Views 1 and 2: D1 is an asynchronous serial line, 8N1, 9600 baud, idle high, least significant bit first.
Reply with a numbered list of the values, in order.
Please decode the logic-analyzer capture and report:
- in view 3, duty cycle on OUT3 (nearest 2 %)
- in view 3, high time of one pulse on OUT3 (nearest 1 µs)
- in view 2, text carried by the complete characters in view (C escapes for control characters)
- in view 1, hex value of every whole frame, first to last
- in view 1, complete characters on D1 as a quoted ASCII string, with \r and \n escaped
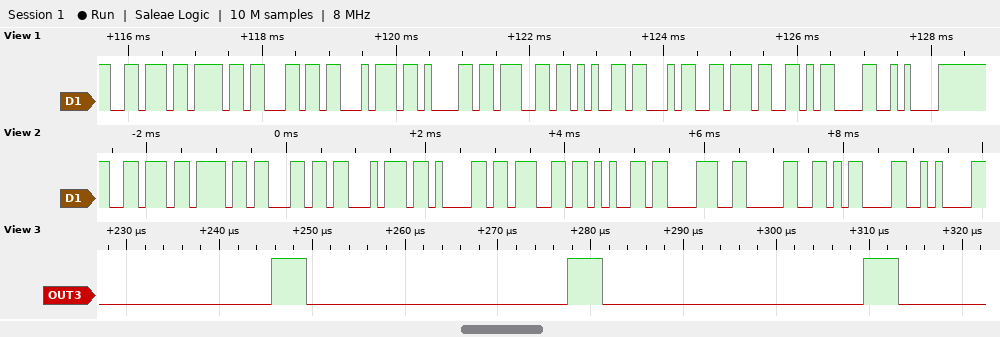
1. 12 %
2. 4 µs
3. "voltage80\r\n"
4. 76 6F 6C 74 61 67 65 34 37 0D 0A
5. "voltage47\r\n"
